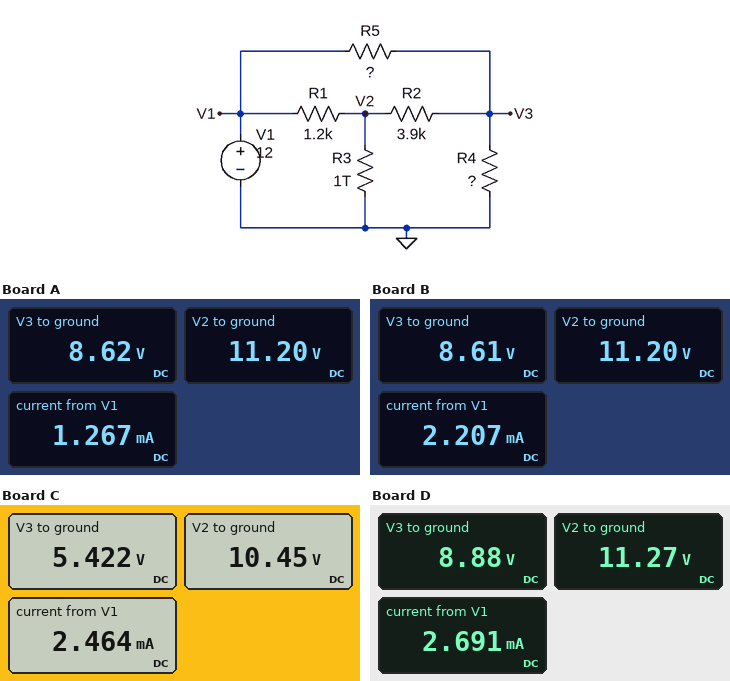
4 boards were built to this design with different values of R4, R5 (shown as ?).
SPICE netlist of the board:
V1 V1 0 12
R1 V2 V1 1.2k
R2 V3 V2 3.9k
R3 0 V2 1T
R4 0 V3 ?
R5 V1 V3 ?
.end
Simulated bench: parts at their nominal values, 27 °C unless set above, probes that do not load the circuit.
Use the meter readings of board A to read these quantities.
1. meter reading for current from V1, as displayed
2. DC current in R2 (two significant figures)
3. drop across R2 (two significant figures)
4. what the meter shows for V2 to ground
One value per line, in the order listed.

1.267 mA
660 µA
2.6 V
11.20 V
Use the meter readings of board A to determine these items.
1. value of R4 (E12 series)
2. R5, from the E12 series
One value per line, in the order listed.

6.8 kΩ
5.6 kΩ
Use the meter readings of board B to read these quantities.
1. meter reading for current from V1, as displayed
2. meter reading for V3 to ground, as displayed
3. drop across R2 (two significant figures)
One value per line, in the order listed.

2.207 mA
8.61 V
2.6 V
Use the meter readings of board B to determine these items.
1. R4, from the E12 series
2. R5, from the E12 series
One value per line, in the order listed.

3.9 kΩ
2.2 kΩ
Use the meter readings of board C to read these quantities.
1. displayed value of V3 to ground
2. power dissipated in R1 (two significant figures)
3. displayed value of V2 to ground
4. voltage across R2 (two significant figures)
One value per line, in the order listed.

5.422 V
2.0 mW
10.45 V
5.0 V
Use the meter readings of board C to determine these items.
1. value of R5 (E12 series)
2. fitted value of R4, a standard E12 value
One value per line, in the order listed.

5.6 kΩ
2.2 kΩ
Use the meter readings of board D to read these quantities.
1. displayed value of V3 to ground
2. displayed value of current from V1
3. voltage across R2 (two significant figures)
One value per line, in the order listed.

8.88 V
2.691 mA
2.4 V
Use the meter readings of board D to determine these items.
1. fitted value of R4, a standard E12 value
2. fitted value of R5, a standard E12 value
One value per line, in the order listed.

3.3 kΩ
1.5 kΩ
